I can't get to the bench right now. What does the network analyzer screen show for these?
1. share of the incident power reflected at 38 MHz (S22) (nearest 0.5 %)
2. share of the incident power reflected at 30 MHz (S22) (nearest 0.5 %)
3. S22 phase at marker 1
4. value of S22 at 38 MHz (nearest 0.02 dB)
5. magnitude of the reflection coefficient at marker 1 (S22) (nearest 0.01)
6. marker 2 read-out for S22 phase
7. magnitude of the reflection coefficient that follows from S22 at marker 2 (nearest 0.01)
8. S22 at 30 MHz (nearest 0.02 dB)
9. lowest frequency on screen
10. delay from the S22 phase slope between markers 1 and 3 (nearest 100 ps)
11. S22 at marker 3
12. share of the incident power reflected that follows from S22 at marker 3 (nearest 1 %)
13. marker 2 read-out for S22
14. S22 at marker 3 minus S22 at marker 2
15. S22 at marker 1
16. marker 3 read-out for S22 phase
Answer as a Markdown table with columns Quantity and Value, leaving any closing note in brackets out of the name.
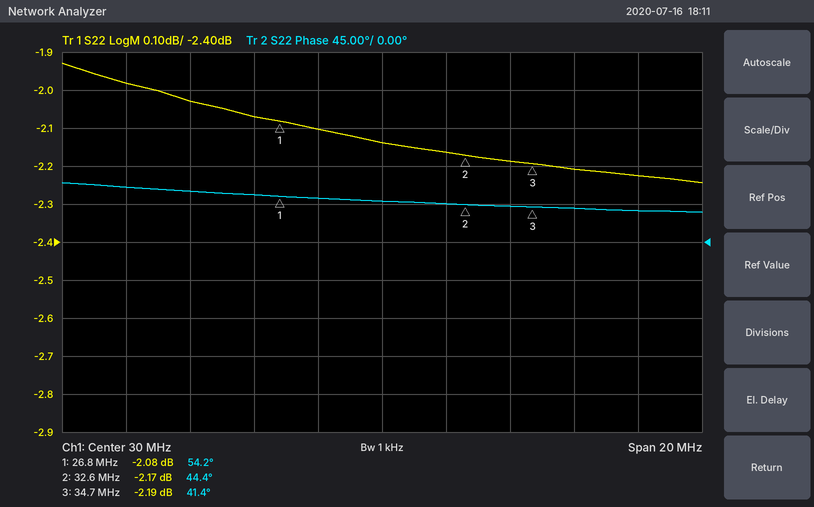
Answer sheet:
| Quantity | Value |
|---|---|
| share of the incident power reflected at 38 MHz (S22) | 60.0 % |
| share of the incident power reflected at 30 MHz (S22) | 61.0 % |
| S22 phase at marker 1 | 54.2° |
| value of S22 at 38 MHz | -2.22 dB |
| magnitude of the reflection coefficient at marker 1 (S22) | 0.79 |
| marker 2 read-out for S22 phase | 44.4° |
| magnitude of the reflection coefficient that follows from S22 at marker 2 | 0.78 |
| S22 at 30 MHz | -2.14 dB |
| lowest frequency on screen | 20 MHz |
| delay from the S22 phase slope between markers 1 and 3 | 4.5 ns |
| S22 at marker 3 | -2.19 dB |
| share of the incident power reflected that follows from S22 at marker 3 | 60 % |
| marker 2 read-out for S22 | -2.17 dB |
| S22 at marker 3 minus S22 at marker 2 | -0.02 dB |
| S22 at marker 1 | -2.08 dB |
| marker 3 read-out for S22 phase | 41.4° |
